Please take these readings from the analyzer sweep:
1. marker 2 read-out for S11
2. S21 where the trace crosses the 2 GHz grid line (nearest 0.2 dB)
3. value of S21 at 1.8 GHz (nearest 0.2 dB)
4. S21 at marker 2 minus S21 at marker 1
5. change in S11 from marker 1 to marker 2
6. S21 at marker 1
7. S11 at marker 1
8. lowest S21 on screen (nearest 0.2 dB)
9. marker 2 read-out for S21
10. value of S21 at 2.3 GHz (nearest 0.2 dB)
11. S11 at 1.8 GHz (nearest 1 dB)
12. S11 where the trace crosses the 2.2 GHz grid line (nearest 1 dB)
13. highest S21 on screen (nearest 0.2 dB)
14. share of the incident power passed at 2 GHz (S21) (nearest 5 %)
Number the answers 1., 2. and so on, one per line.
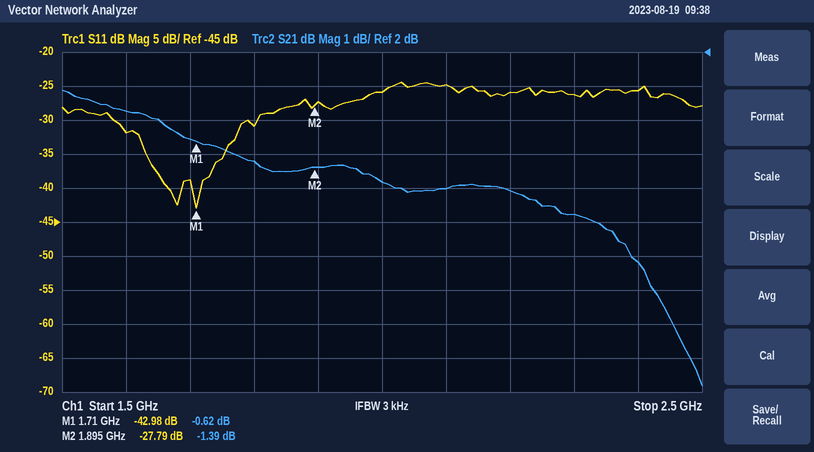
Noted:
1. -27.79 dB
2. -1.8 dB
3. -1.2 dB
4. -0.77 dB
5. 15.19 dB
6. -0.62 dB
7. -42.98 dB
8. -7.8 dB
9. -1.39 dB
10. -2.8 dB
11. -31 dB
12. -26 dB
13. 0.8 dB
14. 65 %
